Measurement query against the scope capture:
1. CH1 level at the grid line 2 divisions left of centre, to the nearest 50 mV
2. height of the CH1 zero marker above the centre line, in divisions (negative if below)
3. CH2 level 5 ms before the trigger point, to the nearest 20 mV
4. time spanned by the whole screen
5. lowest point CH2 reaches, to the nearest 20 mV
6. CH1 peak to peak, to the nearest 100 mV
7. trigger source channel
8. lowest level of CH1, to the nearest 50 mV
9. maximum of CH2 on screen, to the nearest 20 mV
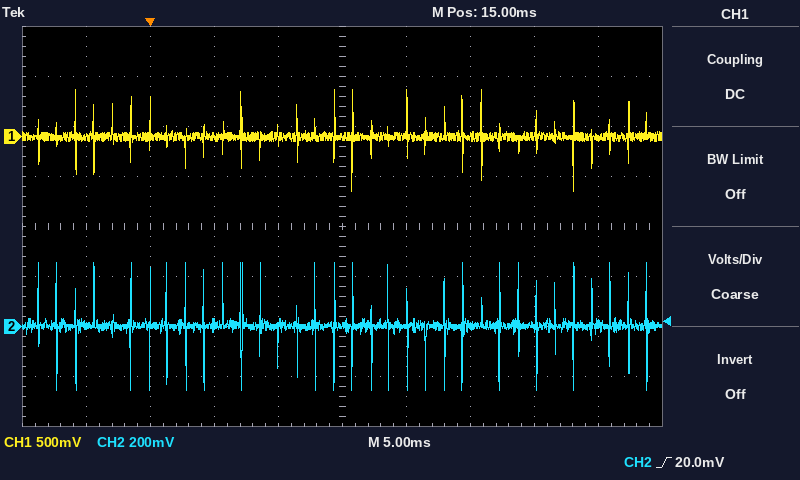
0 mV
+1.8 div
0 mV
50 ms
-260 mV
1.00 V
CH2
-550 mV
260 mV
